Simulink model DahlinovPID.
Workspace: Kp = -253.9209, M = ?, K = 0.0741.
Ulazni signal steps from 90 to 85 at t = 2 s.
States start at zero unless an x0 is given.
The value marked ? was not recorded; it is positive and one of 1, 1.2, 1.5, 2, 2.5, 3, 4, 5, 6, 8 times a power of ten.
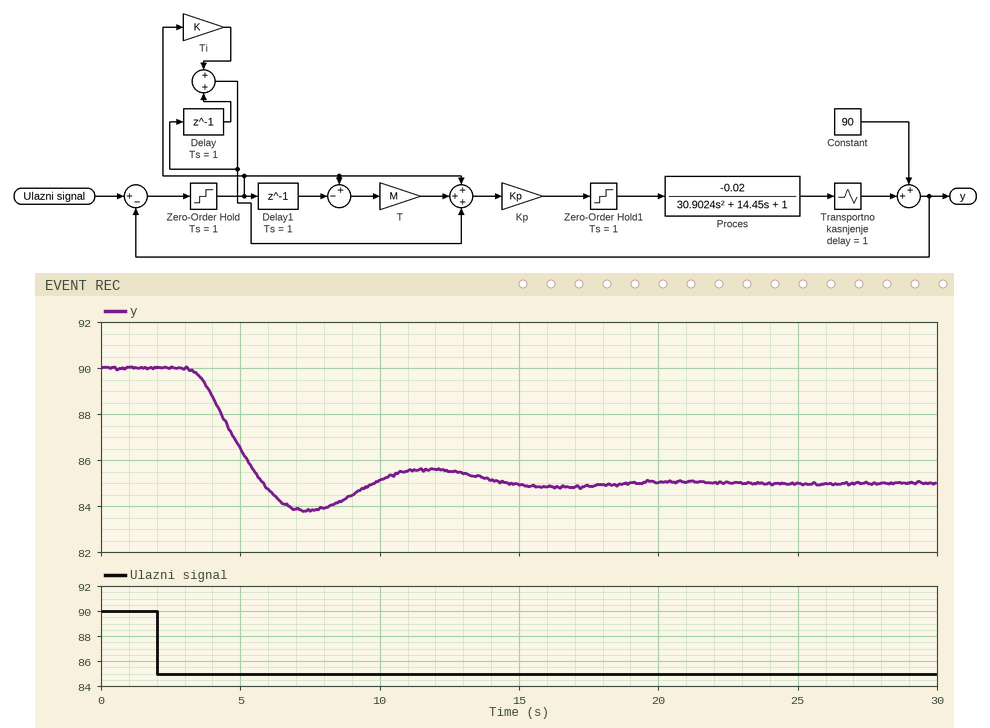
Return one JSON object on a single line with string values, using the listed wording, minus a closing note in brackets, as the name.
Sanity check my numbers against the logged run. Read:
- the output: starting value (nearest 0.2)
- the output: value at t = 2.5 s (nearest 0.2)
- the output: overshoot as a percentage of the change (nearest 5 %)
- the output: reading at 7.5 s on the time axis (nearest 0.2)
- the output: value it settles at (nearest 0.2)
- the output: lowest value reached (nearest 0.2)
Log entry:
{"the output: starting value": "90.0", "the output: value at t = 2.5 s": "90.0", "the output: overshoot as a percentage of the change": "25 %", "the output: reading at 7.5 s on the time axis": "83.8", "the output: value it settles at": "85.0", "the output: lowest value reached": "83.8"}
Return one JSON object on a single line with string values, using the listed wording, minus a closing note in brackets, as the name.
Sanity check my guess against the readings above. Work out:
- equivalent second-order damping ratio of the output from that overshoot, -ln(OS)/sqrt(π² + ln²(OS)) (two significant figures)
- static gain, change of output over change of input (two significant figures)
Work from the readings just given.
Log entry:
{"equivalent second-order damping ratio of the output from that overshoot, -ln(OS)/sqrt(π² + ln²(OS))": "0.40", "static gain, change of output over change of input": "1.0"}
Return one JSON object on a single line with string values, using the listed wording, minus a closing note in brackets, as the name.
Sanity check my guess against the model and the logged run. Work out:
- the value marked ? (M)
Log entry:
{"the value marked ?": "2.5"}
